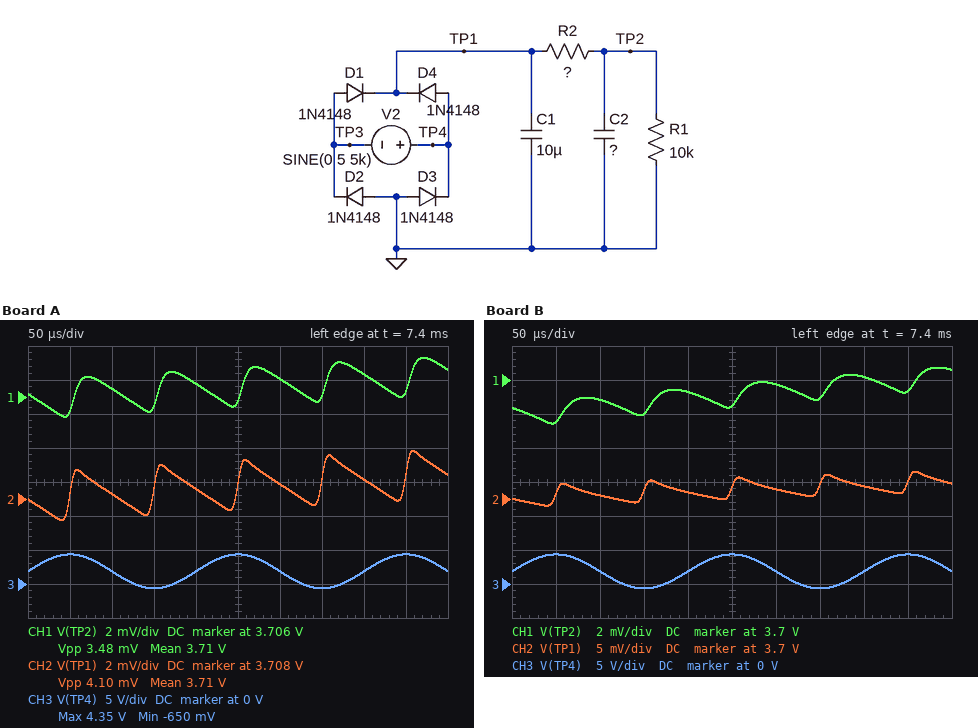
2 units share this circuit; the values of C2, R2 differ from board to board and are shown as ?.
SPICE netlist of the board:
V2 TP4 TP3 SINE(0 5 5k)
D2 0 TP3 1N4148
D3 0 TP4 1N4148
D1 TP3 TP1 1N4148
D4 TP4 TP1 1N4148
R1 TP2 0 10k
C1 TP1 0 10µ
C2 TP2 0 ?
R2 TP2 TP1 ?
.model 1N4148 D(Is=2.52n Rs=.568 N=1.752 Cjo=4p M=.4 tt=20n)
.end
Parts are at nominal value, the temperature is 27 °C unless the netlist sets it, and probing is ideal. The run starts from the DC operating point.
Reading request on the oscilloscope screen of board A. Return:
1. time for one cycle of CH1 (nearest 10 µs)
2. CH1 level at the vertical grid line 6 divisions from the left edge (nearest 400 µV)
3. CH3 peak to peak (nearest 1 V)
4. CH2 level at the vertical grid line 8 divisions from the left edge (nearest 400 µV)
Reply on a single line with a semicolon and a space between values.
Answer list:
100 µs; 3.7072 V; 5 V; 3.7092 V
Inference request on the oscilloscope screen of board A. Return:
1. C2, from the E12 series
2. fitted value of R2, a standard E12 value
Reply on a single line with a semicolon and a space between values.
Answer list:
1.5 µF; 5.6 Ω
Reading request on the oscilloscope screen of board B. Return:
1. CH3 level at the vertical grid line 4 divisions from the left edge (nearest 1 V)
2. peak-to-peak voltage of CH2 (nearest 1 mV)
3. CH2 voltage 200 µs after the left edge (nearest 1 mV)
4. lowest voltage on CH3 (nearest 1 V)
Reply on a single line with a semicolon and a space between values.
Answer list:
2 V; 5 mV; 3.701 V; -1 V
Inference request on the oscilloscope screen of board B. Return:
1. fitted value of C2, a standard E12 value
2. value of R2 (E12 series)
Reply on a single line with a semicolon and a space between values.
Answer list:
4.7 µF; 5.6 Ω
